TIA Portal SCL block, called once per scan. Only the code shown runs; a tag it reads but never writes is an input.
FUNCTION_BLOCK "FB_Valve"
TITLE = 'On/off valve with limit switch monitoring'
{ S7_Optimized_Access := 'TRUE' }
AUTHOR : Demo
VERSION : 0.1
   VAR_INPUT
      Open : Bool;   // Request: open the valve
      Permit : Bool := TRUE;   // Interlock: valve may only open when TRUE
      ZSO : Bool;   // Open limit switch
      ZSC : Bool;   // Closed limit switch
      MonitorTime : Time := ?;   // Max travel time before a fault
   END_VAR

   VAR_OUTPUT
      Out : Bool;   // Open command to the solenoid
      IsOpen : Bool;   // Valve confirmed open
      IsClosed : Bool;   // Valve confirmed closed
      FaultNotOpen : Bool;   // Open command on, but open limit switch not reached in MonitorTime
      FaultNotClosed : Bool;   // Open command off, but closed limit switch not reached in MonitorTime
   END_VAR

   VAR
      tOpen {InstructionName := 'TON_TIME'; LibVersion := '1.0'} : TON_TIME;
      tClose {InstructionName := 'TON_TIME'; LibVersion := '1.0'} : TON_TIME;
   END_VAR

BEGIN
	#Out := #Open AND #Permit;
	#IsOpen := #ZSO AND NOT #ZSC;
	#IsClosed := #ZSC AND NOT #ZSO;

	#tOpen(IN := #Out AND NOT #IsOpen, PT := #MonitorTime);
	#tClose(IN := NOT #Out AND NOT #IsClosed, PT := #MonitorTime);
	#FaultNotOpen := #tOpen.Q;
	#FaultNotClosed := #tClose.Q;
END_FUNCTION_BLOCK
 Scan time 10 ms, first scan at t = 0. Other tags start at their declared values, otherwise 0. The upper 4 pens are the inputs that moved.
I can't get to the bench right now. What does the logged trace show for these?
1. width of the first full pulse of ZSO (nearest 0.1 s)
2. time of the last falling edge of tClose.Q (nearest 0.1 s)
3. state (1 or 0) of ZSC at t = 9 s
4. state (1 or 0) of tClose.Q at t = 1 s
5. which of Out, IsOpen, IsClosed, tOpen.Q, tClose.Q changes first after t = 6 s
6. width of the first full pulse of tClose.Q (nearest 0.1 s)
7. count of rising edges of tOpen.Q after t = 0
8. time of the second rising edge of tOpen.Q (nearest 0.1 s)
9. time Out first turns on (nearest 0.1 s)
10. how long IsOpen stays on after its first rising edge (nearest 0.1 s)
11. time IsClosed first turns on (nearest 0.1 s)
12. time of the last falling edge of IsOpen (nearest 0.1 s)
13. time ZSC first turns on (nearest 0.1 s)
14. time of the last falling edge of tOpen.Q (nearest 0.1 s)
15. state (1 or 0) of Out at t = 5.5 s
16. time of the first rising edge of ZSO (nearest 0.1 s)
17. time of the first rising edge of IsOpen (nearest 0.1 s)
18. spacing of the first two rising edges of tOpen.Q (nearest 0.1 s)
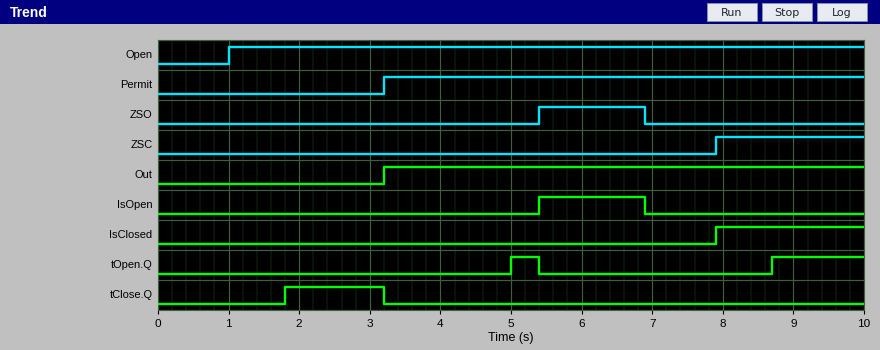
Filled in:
1.5 s
3.2 s
1
0
IsOpen
1.4 s
2
8.7 s
3.2 s
1.5 s
7.9 s
6.9 s
7.9 s
5.4 s
1
5.4 s
5.4 s
3.7 s
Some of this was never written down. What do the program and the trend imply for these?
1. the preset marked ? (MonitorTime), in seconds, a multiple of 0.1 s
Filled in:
1.8 s
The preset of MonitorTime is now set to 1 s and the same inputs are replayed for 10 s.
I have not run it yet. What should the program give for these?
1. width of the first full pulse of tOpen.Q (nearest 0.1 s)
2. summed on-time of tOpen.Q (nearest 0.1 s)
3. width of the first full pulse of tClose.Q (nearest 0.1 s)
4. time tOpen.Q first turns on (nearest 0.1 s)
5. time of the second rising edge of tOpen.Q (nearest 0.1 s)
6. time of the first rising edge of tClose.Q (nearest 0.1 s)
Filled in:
1.2 s
3.3 s
2.2 s
4.2 s
7.9 s
1.0 s
